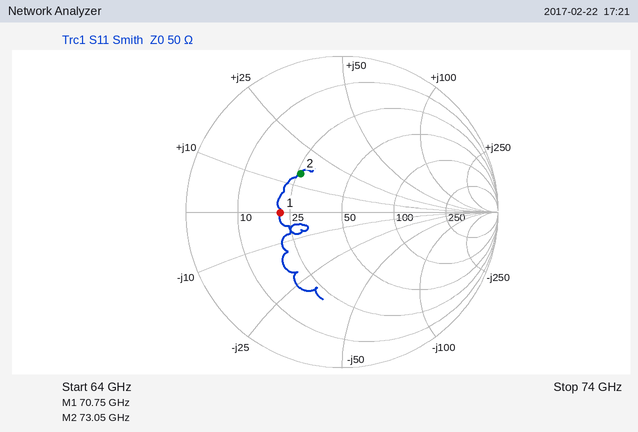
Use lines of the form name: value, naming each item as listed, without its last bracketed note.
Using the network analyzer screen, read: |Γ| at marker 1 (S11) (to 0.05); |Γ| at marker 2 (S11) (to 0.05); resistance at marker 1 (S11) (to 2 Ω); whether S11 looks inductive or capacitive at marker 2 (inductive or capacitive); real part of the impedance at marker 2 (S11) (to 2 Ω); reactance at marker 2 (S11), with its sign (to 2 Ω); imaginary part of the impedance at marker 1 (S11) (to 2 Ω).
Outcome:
|Γ| at marker 1 (S11): 0.40
|Γ| at marker 2 (S11): 0.35
resistance at marker 1 (S11): 22 Ω
whether S11 looks inductive or capacitive at marker 2: inductive
real part of the impedance at marker 2 (S11): 26 Ω
reactance at marker 2 (S11), with its sign: +14 Ω
imaginary part of the impedance at marker 1 (S11): 0 Ω
